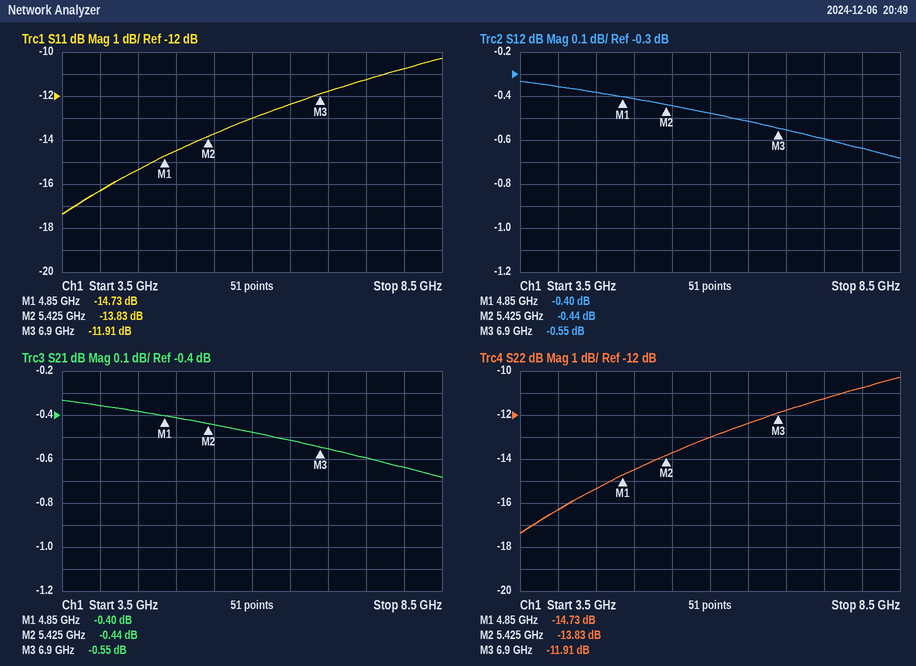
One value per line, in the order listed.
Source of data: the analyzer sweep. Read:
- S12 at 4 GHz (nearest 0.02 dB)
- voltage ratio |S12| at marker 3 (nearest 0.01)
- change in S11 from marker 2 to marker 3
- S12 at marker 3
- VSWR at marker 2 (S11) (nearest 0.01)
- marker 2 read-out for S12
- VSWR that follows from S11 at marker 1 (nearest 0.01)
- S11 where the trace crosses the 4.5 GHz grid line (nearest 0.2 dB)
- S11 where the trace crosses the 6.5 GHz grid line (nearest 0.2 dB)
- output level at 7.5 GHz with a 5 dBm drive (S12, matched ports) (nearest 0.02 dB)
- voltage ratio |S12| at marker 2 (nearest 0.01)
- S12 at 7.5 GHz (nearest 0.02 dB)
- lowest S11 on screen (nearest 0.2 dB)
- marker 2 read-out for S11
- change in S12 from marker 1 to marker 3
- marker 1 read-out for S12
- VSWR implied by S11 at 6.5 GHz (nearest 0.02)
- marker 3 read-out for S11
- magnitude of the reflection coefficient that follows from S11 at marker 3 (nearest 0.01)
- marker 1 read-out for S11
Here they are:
-0.36 dB
0.94
1.92 dB
-0.55 dB
1.51
-0.44 dB
1.45
-15.4 dB
-12.4 dB
4.40 dBm
0.95
-0.60 dB
-17.4 dB
-13.83 dB
-0.15 dB
-0.40 dB
1.64
-11.91 dB
0.25
-14.73 dB
